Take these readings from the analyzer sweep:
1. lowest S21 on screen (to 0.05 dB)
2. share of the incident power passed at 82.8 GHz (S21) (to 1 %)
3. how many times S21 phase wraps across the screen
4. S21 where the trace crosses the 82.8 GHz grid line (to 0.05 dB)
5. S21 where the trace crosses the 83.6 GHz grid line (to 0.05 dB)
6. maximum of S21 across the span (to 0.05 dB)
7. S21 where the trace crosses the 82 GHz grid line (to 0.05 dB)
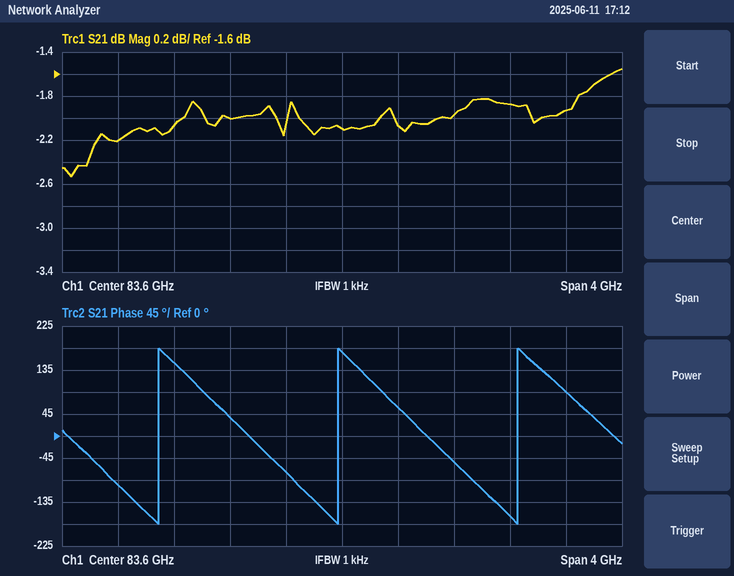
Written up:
-2.55 dB
63 %
3
-2.00 dB
-2.10 dB
-1.55 dB
-2.20 dB
